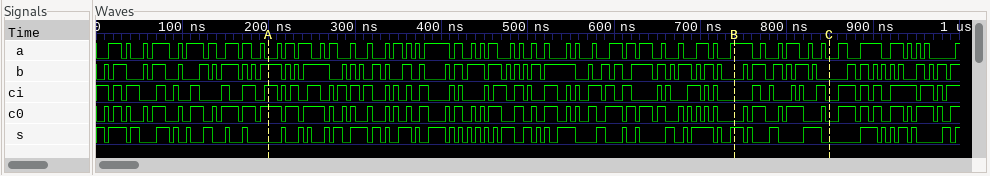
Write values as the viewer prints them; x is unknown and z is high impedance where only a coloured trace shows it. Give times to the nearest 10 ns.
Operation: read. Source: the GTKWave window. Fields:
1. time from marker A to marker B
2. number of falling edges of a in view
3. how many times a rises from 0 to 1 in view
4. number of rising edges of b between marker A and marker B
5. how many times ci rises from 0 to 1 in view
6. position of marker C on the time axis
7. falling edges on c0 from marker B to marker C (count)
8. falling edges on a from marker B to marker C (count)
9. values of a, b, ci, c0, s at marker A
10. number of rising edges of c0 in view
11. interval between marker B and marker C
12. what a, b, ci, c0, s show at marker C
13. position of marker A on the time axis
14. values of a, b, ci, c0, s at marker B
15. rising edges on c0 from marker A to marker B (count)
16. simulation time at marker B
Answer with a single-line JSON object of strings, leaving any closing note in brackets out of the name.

{"time from marker A to marker B": "540 ns", "number of falling edges of a in view": "52", "how many times a rises from 0 to 1 in view": "53", "number of rising edges of b between marker A and marker B": "29", "how many times ci rises from 0 to 1 in view": "48", "position of marker C on the time axis": "850 ns", "falling edges on c0 from marker B to marker C": "5", "falling edges on a from marker B to marker C": "6", "values of a, b, ci, c0, s at marker A": "a=0, b=1, ci=1, c0=1, s=0", "number of rising edges of c0 in view": "54", "interval between marker B and marker C": "110 ns", "what a, b, ci, c0, s show at marker C": "a=0, b=0, ci=0, c0=0, s=0", "position of marker A on the time axis": "200 ns", "values of a, b, ci, c0, s at marker B": "a=1, b=0, ci=0, c0=0, s=1", "rising edges on c0 from marker A to marker B": "30", "simulation time at marker B": "740 ns"}
